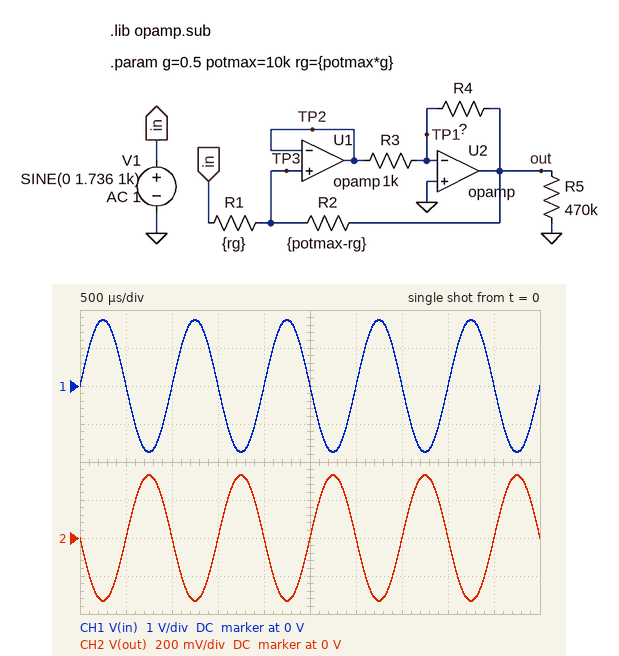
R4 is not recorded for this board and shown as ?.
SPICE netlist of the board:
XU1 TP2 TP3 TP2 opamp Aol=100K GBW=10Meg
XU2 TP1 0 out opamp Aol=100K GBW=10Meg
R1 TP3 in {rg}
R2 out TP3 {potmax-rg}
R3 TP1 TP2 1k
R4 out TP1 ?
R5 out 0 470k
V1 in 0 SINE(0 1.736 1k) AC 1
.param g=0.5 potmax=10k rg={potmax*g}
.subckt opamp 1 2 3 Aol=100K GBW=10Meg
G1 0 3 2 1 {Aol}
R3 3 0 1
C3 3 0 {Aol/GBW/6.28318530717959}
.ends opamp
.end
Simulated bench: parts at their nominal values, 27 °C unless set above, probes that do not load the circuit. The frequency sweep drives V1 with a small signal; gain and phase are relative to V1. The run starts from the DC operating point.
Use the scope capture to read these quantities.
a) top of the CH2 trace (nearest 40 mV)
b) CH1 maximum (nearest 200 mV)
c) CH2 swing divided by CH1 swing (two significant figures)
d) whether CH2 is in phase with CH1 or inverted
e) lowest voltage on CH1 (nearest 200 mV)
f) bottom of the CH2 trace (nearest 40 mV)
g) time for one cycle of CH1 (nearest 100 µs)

320 mV
1.8 V
0.19
inverted
-1.8 V
-320 mV
1.0 ms
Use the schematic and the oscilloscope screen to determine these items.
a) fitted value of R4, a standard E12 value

470 Ω
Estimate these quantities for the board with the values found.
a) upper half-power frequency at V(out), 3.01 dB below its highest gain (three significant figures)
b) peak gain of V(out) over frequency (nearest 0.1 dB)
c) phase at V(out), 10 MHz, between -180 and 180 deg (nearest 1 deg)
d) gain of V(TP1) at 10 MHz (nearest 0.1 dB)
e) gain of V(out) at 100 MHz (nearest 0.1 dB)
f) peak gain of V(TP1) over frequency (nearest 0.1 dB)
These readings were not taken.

6.67 MHz
-14.4 dB
85 deg
-20.5 dB
-56.0 dB
-20.4 dB
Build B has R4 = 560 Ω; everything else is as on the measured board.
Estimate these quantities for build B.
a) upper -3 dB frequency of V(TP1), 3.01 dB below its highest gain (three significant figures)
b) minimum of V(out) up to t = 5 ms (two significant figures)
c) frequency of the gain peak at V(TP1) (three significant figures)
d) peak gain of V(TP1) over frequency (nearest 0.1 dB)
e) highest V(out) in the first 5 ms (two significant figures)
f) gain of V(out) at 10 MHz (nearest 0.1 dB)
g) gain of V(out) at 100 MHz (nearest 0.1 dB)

20.4 MHz
-380 mV
9.06 MHz
-19.2 dB
380 mV
-19.3 dB
-55.0 dB
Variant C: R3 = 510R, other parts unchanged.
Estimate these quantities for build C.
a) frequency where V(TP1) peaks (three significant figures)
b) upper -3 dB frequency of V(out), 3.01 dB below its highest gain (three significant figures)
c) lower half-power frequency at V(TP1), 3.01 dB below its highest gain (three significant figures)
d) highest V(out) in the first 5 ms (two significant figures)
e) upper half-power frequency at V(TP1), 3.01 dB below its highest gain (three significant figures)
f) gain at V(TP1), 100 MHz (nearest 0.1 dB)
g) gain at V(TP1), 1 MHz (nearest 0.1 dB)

8.72 MHz
6.79 MHz
3.97 MHz
550 mV
19.2 MHz
-32.4 dB
-30.1 dB
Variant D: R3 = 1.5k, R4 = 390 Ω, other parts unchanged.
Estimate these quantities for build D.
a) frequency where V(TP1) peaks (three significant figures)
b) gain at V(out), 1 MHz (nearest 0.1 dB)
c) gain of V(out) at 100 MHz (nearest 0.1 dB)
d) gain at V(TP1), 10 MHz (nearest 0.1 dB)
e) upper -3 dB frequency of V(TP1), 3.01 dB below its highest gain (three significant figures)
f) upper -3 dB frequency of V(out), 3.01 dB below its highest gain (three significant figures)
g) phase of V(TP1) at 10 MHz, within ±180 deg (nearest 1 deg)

9.47 MHz
-18.9 dB
-59.8 dB
-24.8 dB
22.0 MHz
6.58 MHz
-3 deg
